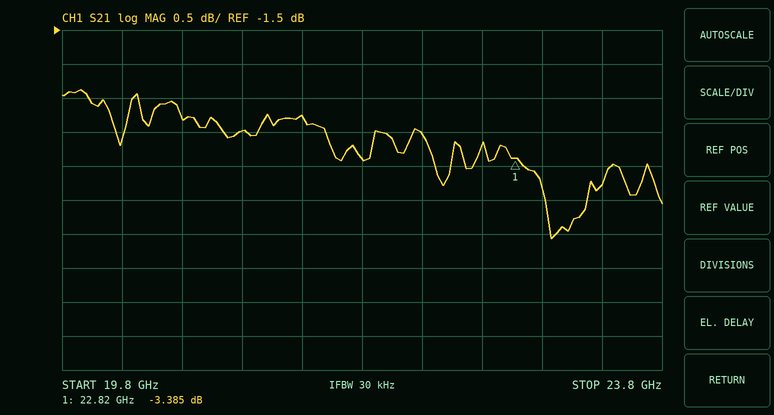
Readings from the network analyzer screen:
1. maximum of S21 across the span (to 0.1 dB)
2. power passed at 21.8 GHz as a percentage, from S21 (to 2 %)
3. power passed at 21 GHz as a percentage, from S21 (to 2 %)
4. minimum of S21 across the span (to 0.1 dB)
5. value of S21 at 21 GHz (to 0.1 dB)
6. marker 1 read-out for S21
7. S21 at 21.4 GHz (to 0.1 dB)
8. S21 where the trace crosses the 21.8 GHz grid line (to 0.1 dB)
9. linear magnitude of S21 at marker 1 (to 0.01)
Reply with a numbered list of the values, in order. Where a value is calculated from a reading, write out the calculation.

1. -2.4 dB
2. 10^(-3.4/10) ≈ 46 %
3. 10^(-3/10) ≈ 50 %
4. -4.6 dB
5. -3.0 dB
6. -3.385 dB
7. -2.8 dB
8. -3.4 dB
9. 10^(-3.385/20) ≈ 0.68
